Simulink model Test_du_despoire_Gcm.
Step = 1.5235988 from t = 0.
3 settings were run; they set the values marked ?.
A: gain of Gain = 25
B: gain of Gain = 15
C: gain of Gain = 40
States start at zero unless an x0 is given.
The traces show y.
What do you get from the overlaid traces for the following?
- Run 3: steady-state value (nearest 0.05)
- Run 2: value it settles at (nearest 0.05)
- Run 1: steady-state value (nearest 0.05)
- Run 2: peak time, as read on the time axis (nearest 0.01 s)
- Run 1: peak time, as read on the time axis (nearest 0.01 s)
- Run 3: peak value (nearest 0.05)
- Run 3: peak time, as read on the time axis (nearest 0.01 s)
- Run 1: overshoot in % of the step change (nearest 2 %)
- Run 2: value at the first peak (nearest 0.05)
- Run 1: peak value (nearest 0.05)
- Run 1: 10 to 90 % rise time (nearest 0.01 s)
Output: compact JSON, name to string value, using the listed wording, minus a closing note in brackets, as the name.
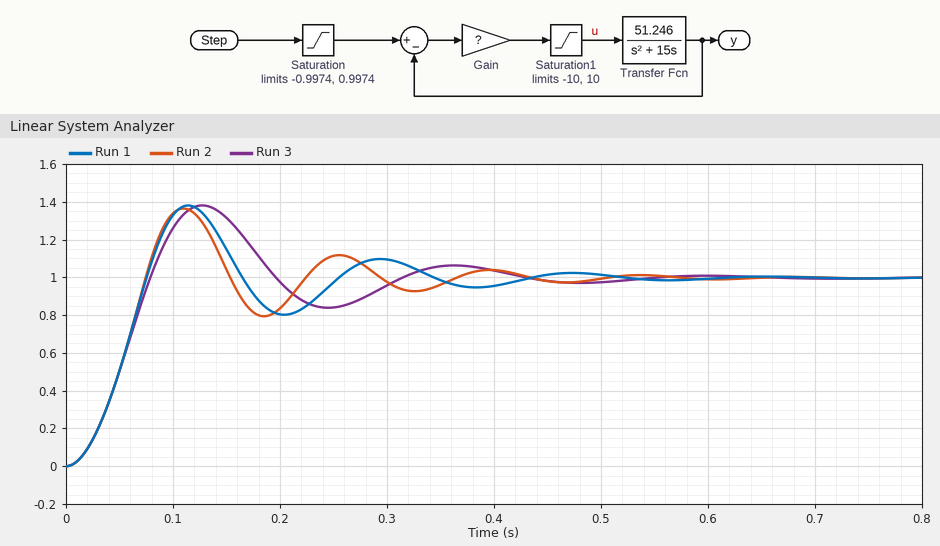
{"Run 3: steady-state value": "1.00", "Run 2: value it settles at": "1.00", "Run 1: steady-state value": "1.00", "Run 2: peak time, as read on the time axis": "0.11 s", "Run 1: peak time, as read on the time axis": "0.11 s", "Run 3: peak value": "1.40", "Run 3: peak time, as read on the time axis": "0.13 s", "Run 1: overshoot in % of the step change": "38 %", "Run 2: value at the first peak": "1.35", "Run 1: peak value": "1.40", "Run 1: 10 to 90 % rise time": "0.05 s"}
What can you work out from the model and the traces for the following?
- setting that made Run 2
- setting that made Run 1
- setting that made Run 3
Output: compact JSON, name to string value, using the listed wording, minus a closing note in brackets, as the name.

{"setting that made Run 2": "C", "setting that made Run 1": "A", "setting that made Run 3": "B"}
